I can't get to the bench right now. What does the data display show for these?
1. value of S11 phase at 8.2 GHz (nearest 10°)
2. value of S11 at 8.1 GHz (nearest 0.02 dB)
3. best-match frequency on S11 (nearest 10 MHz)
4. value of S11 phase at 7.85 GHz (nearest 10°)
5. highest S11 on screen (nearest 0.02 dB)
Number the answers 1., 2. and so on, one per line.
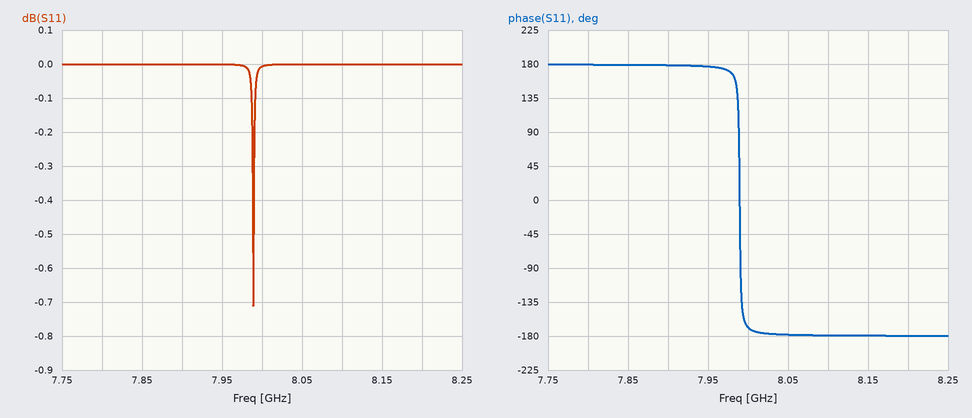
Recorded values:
1. -180°
2. 0.00 dB
3. 7.99 GHz
4. 180°
5. 0.00 dB
